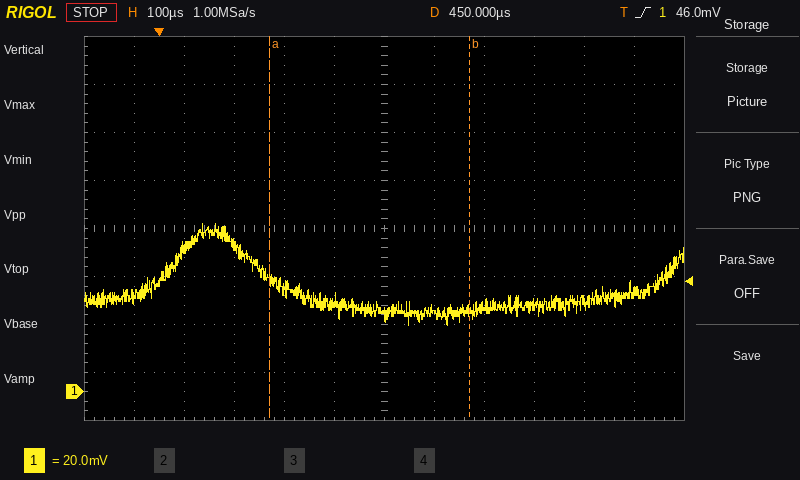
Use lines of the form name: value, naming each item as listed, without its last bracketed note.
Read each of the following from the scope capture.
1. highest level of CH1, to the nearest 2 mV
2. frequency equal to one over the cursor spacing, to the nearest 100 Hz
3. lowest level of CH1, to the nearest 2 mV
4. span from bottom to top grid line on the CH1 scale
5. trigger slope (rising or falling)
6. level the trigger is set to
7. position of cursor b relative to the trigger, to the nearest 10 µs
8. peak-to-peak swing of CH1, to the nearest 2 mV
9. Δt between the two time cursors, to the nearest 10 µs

highest level of CH1, to the nearest 2 mV: 70 mV
frequency equal to one over the cursor spacing, to the nearest 100 Hz: 2.5 kHz
lowest level of CH1, to the nearest 2 mV: 28 mV
span from bottom to top grid line on the CH1 scale: 160 mV
trigger slope: rising
level the trigger is set to: 46.0 mV
position of cursor b relative to the trigger, to the nearest 10 µs: +620 µs
peak-to-peak swing of CH1, to the nearest 2 mV: 42 mV
Δt between the two time cursors, to the nearest 10 µs: 400 µs
